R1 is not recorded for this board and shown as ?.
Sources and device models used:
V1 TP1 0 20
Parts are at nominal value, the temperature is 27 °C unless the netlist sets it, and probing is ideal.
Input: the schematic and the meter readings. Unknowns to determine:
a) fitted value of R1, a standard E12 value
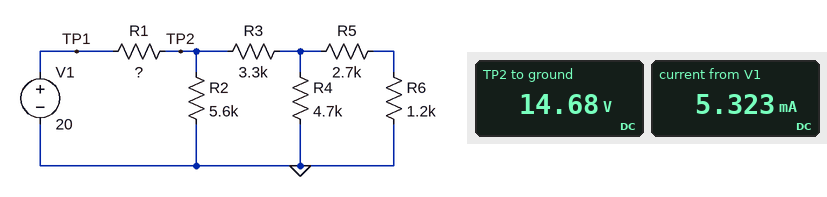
1 kΩ
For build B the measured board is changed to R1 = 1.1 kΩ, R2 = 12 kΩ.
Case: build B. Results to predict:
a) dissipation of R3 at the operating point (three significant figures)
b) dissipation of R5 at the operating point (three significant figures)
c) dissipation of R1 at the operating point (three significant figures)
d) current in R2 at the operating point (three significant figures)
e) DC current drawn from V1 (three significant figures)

26.7 mW
6.53 mW
18.8 mW
1.29 mA
4.13 mA
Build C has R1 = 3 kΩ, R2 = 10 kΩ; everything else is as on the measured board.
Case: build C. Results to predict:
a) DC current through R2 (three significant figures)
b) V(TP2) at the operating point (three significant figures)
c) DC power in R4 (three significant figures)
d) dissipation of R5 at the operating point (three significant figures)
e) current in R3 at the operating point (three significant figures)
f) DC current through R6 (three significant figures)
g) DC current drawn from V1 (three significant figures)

1.08 mA
10.8 V
3.82 mW
3.19 mW
1.99 mA
1.09 mA
3.07 mA
